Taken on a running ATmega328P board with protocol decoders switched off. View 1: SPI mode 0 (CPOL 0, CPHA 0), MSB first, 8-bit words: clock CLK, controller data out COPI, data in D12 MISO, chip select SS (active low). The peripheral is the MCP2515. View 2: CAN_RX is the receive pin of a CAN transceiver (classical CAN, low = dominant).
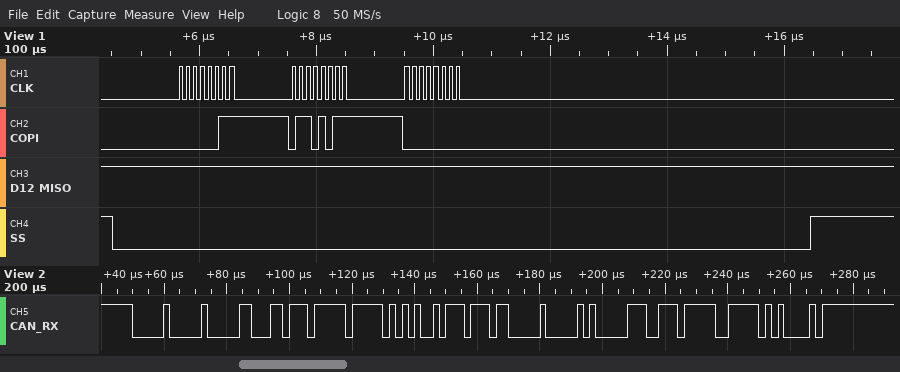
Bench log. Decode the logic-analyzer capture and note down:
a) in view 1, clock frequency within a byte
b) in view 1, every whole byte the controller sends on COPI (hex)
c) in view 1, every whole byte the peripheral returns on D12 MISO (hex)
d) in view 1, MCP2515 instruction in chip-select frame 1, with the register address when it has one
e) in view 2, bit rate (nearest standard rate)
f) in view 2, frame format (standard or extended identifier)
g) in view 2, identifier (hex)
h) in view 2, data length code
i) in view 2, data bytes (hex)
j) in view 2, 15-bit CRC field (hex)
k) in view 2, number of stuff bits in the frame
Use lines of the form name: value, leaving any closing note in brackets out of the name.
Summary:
in view 1, clock frequency within a byte: 8 MHz
in view 1, every whole byte the controller sends on COPI: 0x03 0x6B 0x00
in view 1, every whole byte the peripheral returns on D12 MISO: 0xFF 0xFF 0xFF
in view 1, MCP2515 instruction in chip-select frame 1, with the register address when it has one: READ 0x6B
in view 2, bit rate: 500 kbit/s
in view 2, frame format: standard
in view 2, identifier: 0x000
in view 2, data length code: 8
in view 2, data bytes: DD FF D4 BB B0 01 06 77
in view 2, 15-bit CRC field: 0x6FD0
in view 2, number of stuff bits in the frame: 10
